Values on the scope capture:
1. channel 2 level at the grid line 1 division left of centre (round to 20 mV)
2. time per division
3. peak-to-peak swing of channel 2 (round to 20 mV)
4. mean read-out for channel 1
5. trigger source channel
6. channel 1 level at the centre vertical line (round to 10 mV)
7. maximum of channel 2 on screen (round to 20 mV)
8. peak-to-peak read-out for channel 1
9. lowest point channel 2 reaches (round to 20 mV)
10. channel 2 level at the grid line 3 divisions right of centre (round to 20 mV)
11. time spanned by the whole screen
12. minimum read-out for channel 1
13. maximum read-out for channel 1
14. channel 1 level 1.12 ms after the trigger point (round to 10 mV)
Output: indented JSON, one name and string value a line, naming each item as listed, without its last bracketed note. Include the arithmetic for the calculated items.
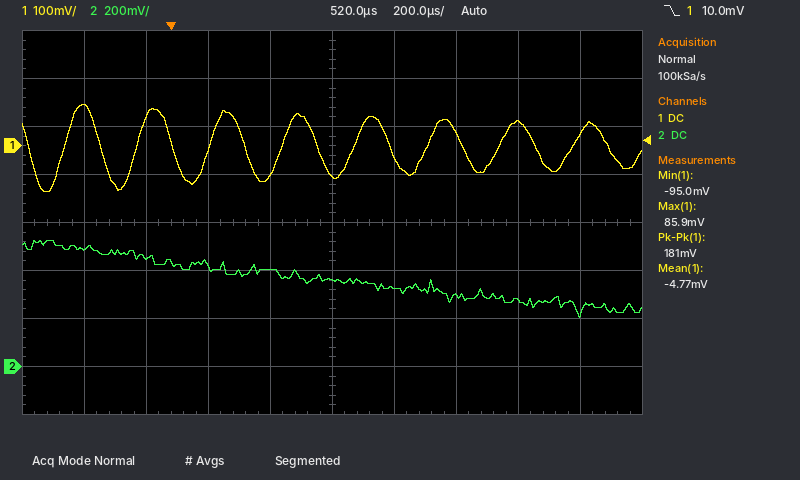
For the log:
{
  "channel 2 level at the grid line 1 division left of centre": "400 mV",
  "time per division": "200 µs",
  "peak-to-peak swing of channel 2": "520 mV − (200 mV) = 320 mV",
  "mean read-out for channel 1": "-4.77 mV",
  "trigger source channel": "channel 1",
  "channel 1 level at the centre vertical line": "-60 mV",
  "maximum of channel 2 on screen": "520 mV",
  "peak-to-peak read-out for channel 1": "181 mV",
  "lowest point channel 2 reaches": "200 mV",
  "channel 2 level at the grid line 3 divisions right of centre": "280 mV",
  "time spanned by the whole screen": "2 ms",
  "minimum read-out for channel 1": "-95.0 mV",
  "maximum read-out for channel 1": "85.9 mV",
  "channel 1 level 1.12 ms after the trigger point": "50 mV"
}
